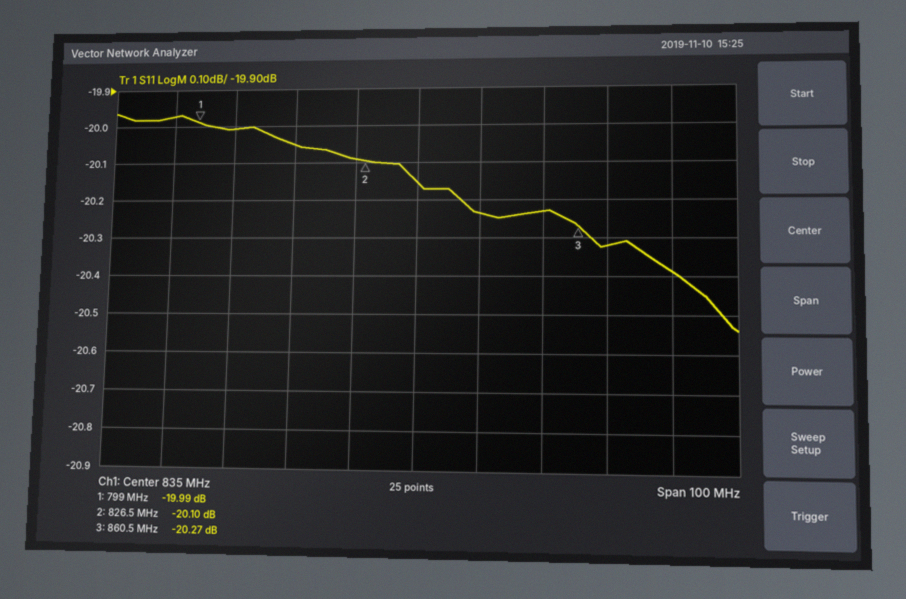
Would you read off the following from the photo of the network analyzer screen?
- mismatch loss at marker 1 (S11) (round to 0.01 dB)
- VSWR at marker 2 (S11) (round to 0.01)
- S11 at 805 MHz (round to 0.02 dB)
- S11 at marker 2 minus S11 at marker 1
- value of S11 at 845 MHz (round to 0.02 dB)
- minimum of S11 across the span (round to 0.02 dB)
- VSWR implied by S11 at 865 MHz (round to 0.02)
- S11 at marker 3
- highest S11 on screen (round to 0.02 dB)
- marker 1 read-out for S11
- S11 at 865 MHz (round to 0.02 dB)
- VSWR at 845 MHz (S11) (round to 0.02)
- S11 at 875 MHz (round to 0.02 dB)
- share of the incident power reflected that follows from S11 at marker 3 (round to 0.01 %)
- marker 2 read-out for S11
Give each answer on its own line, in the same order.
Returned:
0.04 dB
1.22
-20.00 dB
-0.11 dB
-20.24 dB
-20.54 dB
1.22
-20.27 dB
-19.96 dB
-19.99 dB
-20.32 dB
1.22
-20.38 dB
0.94 %
-20.10 dB
